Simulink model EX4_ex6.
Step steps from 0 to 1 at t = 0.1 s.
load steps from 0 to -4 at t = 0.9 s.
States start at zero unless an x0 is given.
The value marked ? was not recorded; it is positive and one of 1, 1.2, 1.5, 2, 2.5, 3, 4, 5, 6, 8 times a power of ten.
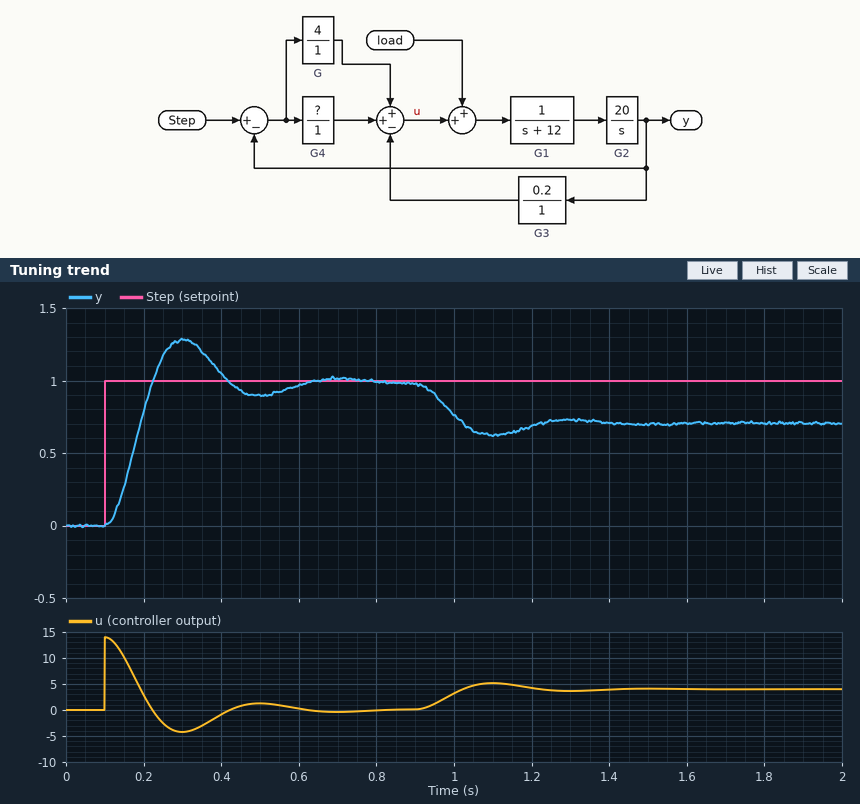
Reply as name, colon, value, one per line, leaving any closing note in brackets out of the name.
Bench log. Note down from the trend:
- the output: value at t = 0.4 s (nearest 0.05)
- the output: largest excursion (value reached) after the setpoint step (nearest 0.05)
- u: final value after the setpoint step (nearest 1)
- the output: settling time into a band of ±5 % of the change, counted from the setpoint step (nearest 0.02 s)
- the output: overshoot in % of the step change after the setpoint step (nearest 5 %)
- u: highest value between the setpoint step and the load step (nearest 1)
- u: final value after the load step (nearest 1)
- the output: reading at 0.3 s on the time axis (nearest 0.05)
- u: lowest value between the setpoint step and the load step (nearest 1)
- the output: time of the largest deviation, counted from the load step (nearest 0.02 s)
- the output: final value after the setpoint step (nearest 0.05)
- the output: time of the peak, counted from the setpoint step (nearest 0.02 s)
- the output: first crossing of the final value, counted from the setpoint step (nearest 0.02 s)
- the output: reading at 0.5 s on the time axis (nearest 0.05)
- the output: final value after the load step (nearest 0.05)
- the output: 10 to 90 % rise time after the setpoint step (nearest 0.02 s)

the output: value at t = 0.4 s: 1.05
the output: largest excursion (value reached) after the setpoint step: 1.30
u: final value after the setpoint step: 0
the output: settling time into a band of ±5 % of the change, counted from the setpoint step: 0.46 s
the output: overshoot in % of the step change after the setpoint step: 30 %
u: highest value between the setpoint step and the load step: 14
u: final value after the load step: 4
the output: reading at 0.3 s on the time axis: 1.30
u: lowest value between the setpoint step and the load step: -4
the output: time of the largest deviation, counted from the load step: 0.20 s
the output: final value after the setpoint step: 1.00
the output: time of the peak, counted from the setpoint step: 0.20 s
the output: first crossing of the final value, counted from the setpoint step: 0.12 s
the output: reading at 0.5 s on the time axis: 0.90
the output: final value after the load step: 0.70
the output: 10 to 90 % rise time after the setpoint step: 0.08 s
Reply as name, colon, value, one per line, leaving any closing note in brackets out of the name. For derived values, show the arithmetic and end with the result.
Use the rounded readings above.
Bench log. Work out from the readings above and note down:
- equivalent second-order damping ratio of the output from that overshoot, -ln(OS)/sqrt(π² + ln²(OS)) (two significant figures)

equivalent second-order damping ratio of the output from that overshoot, -ln(OS)/sqrt(π² + ln²(OS)): ln(0.3) = -1.204; 1.204 / sqrt(9.870 + 1.450) = 0.36
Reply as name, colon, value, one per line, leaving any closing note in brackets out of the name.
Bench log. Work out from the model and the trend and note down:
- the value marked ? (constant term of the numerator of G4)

the value marked ?: 10
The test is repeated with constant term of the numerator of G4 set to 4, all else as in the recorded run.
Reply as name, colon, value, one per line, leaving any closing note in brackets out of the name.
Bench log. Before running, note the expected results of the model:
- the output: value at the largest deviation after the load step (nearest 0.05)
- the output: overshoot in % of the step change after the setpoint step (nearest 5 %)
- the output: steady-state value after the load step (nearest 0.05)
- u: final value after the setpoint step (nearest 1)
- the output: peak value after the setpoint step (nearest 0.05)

the output: value at the largest deviation after the load step: 0.40
the output: overshoot in % of the step change after the setpoint step: 20 %
the output: steady-state value after the load step: 0.50
u: final value after the setpoint step: 0
the output: peak value after the setpoint step: 1.15
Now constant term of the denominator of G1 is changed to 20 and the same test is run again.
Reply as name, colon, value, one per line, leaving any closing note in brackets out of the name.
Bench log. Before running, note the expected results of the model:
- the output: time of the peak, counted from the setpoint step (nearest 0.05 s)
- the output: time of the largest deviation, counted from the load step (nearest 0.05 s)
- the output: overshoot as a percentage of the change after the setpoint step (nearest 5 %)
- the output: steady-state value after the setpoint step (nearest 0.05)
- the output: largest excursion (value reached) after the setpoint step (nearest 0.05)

the output: time of the peak, counted from the setpoint step: 0.25 s
the output: time of the largest deviation, counted from the load step: 0.25 s
the output: overshoot as a percentage of the change after the setpoint step: 10 %
the output: steady-state value after the setpoint step: 1.00
the output: largest excursion (value reached) after the setpoint step: 1.10
